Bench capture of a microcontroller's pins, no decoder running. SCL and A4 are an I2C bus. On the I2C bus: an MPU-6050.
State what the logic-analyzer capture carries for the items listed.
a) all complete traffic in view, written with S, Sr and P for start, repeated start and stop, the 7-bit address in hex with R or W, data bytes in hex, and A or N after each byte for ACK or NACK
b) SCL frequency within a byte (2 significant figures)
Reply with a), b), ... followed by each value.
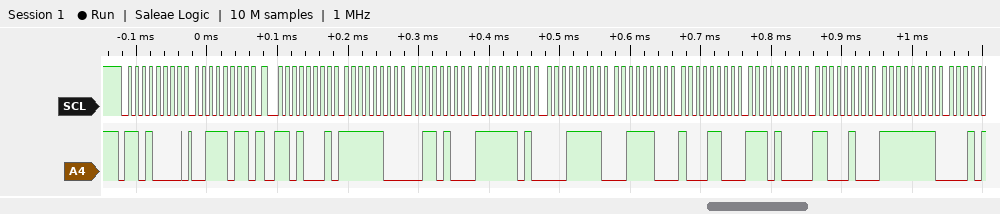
a) S 68W A 3B A Sr 68R A FC A 34 A FD A 1F A 3C A 8C A E8 A C4 A FF A
b) 100 kHz
